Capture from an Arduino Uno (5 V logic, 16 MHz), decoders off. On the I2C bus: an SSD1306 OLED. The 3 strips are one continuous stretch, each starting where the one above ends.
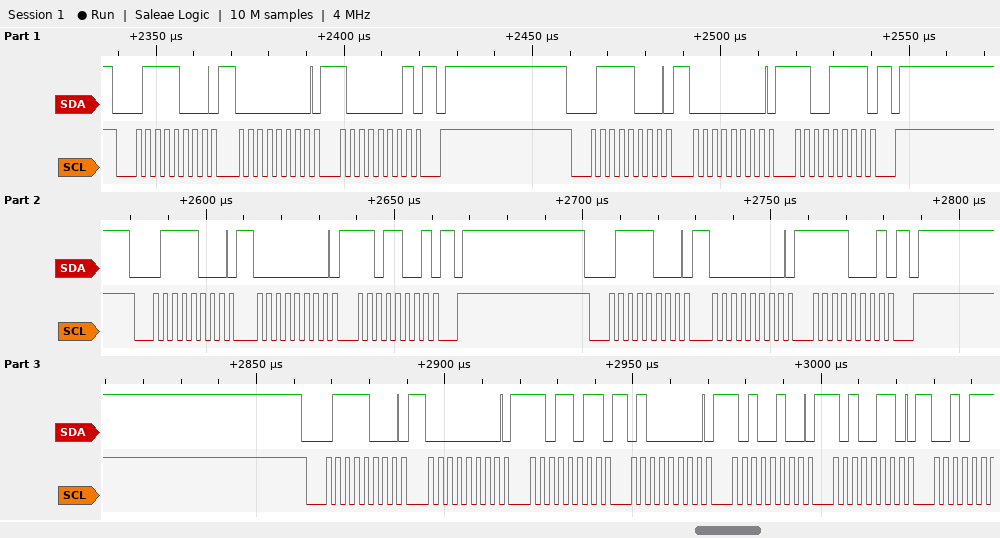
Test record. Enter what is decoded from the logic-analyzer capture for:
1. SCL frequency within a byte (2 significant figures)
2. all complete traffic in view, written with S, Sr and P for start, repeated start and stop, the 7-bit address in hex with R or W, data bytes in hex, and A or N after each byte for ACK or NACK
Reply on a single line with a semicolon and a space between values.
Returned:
400 kHz; S 3CW A 00 A 81 A P S 3CW A 00 A CF A P S 3CW A 00 A D9 A P S 3CW A 00 A F1 A P S 3CW A 00 A DB A 40 A A4 A A6 A
